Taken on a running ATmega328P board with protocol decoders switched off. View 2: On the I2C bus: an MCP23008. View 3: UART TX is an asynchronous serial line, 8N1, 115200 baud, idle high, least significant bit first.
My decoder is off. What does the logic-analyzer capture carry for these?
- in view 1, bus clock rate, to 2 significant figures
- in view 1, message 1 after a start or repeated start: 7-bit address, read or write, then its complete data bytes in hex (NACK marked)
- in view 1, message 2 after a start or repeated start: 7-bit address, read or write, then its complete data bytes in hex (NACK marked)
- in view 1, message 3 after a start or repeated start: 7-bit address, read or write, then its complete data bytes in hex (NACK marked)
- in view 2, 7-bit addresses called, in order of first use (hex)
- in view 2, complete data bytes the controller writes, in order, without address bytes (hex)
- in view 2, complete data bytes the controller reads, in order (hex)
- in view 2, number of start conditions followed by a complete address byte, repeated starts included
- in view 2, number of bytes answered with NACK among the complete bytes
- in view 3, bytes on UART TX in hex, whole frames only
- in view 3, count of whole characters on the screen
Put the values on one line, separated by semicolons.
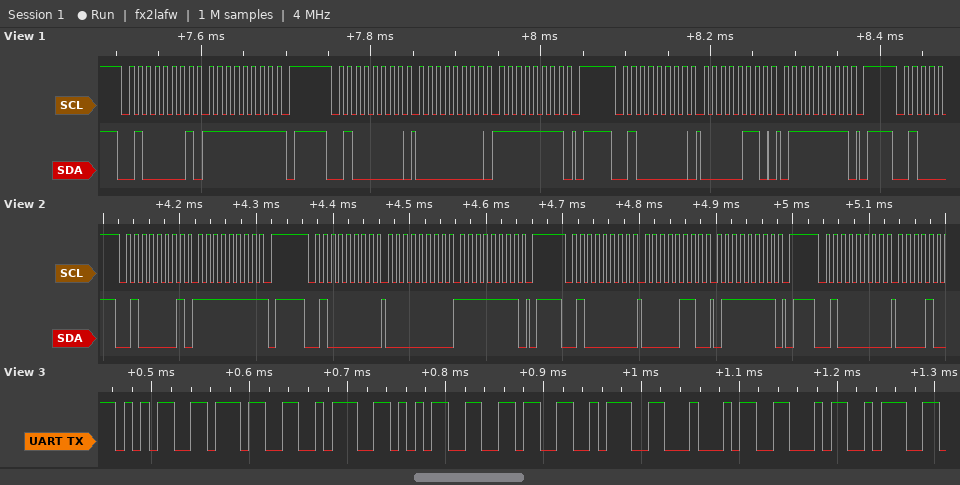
100 kHz; 0x20 read: FF NACK; 0x20 write: 00 FF; 0x20 write: 06 7F; 0x20; 00 FF 06 7F; FF; 4; 1; 35 37 3A 35 36 3A 44 46 3A; 9
